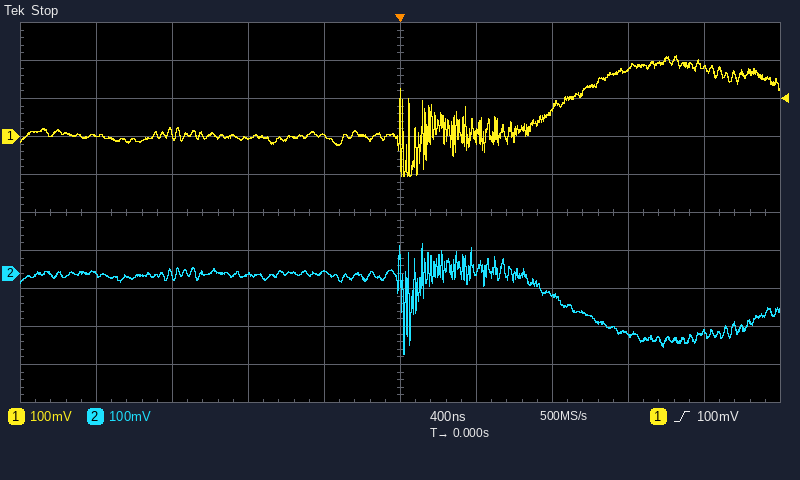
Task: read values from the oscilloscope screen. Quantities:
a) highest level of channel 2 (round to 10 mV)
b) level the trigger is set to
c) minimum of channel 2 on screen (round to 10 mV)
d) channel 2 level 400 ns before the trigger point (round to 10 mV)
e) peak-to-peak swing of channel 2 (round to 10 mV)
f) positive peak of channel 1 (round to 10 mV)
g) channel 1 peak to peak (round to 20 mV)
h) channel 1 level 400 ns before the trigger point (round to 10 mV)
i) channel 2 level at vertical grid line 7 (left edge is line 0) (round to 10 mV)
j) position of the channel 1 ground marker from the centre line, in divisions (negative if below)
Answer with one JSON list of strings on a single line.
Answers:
["80 mV", "100 mV", "-210 mV", "0 mV", "290 mV", "210 mV", "320 mV", "0 mV", "-60 mV", "+2.0 div"]
